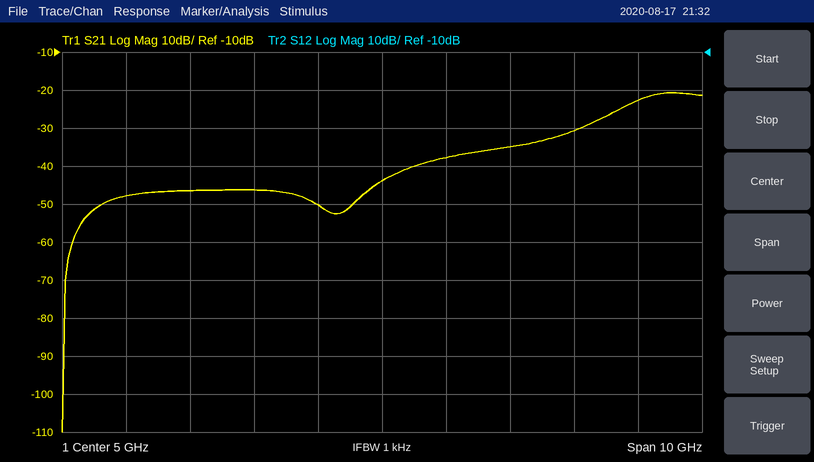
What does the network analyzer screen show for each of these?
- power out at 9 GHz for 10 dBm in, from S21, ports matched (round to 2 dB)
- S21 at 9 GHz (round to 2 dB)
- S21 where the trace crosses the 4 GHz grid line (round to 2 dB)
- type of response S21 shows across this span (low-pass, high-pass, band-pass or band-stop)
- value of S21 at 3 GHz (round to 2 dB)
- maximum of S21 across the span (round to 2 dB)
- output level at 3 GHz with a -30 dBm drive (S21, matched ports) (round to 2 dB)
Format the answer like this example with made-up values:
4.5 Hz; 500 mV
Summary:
-12 dBm; -22 dB; -50 dB; high-pass; -46 dB; -20 dB; -76 dBm
